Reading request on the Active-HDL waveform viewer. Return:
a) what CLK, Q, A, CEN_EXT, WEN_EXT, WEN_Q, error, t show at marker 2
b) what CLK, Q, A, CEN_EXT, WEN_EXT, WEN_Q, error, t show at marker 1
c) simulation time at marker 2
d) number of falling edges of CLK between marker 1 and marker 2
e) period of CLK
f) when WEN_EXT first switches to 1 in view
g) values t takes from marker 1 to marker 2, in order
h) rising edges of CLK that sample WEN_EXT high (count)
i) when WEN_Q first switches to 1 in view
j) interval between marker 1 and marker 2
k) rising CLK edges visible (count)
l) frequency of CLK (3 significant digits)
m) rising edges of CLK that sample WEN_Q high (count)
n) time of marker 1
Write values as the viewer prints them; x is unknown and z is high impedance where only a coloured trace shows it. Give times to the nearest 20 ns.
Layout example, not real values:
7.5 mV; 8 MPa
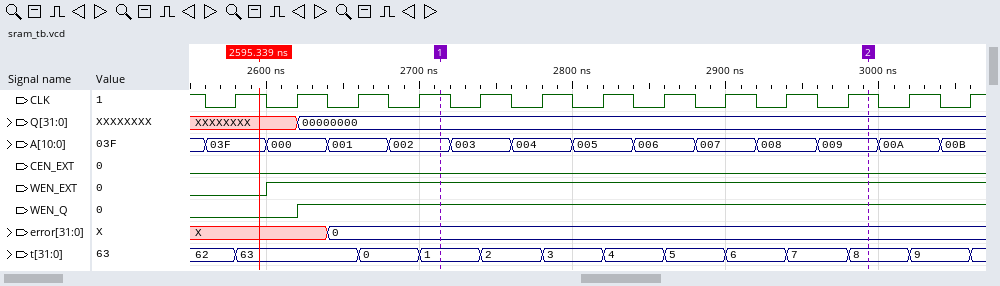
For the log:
CLK=1, Q=00000000, A=009, CEN_EXT=0, WEN_EXT=1, WEN_Q=1, error=0, t=8; CLK=1, Q=00000000, A=002, CEN_EXT=0, WEN_EXT=1, WEN_Q=1, error=0, t=1; 3000 ns; 7; 40 ns; 2600 ns; 1, 2, 3, 4, 5, 6, 7, 8; 12; 2620 ns; 280 ns; 13; 25.0 MHz; 11; 2720 ns
